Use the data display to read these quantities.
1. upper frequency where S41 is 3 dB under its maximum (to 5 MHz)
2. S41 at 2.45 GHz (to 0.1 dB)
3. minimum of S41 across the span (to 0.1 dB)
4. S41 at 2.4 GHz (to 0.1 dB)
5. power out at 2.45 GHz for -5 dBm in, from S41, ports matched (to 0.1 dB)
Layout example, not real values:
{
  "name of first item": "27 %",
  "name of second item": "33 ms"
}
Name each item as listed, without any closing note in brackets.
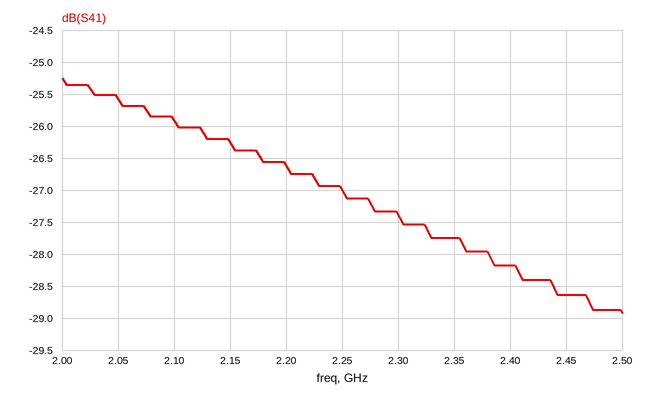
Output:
{
  "upper frequency where S41 is 3 dB under its maximum": "2.405 GHz",
  "S41 at 2.45 GHz": "-28.6 dB",
  "minimum of S41 across the span": "-28.9 dB",
  "S41 at 2.4 GHz": "-28.2 dB",
  "power out at 2.45 GHz for -5 dBm in, from S41, ports matched": "-33.6 dBm"
}
